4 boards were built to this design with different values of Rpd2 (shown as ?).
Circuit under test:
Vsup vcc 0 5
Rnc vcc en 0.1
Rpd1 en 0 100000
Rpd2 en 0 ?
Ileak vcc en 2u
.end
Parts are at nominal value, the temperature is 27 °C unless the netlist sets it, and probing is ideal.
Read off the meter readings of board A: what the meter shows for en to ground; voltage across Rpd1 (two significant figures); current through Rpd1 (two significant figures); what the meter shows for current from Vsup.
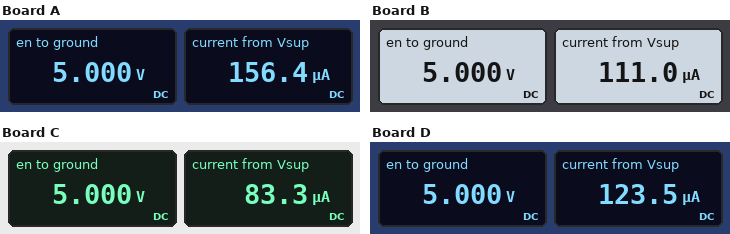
5.000 V
5.0 V
50 µA
156.4 µA
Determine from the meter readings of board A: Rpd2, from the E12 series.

47 kΩ
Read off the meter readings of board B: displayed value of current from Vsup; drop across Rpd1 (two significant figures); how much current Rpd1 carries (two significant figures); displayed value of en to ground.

111.0 µA
5.0 V
50 µA
5.000 V
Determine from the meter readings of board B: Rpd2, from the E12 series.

82 kΩ
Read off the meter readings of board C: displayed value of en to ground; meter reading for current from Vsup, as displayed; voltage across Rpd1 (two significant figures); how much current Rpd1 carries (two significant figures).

5.000 V
83.3 µA
5.0 V
50 µA
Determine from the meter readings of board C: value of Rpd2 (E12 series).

150 kΩ
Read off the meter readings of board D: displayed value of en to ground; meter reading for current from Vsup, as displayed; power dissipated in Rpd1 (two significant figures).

5.000 V
123.5 µA
250 µW
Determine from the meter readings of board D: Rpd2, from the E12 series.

68 kΩ
